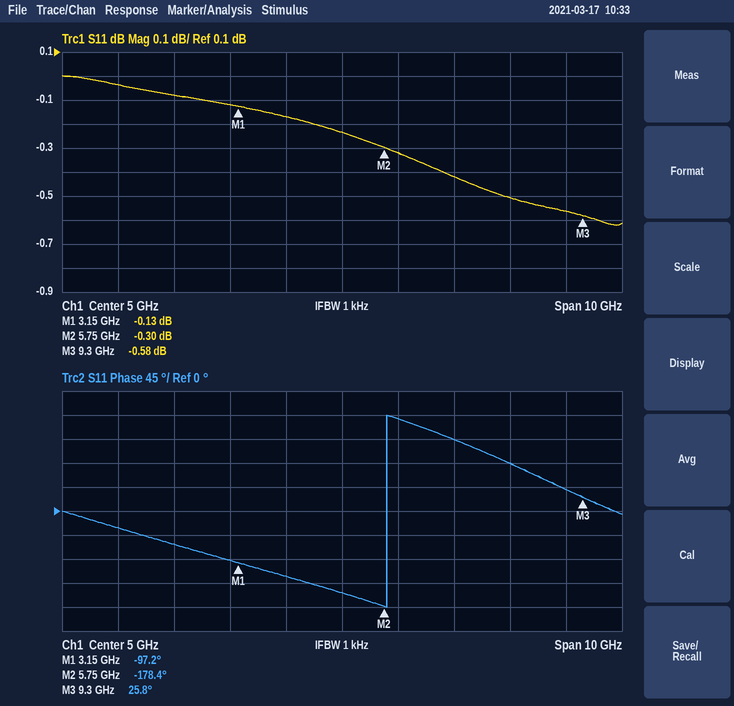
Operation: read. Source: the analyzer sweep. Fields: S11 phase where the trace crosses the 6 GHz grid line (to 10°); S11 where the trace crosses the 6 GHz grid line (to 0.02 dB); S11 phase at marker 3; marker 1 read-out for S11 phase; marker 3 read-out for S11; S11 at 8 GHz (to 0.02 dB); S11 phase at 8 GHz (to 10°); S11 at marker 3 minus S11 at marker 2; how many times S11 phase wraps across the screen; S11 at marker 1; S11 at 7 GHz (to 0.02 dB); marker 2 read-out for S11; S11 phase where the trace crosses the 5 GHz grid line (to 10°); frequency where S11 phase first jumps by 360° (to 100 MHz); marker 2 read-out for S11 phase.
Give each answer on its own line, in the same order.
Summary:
170°
-0.32 dB
25.8°
-97.2°
-0.58 dB
-0.50 dB
90°
-0.28 dB
1
-0.13 dB
-0.42 dB
-0.30 dB
-150°
5.8 GHz
-178.4°
